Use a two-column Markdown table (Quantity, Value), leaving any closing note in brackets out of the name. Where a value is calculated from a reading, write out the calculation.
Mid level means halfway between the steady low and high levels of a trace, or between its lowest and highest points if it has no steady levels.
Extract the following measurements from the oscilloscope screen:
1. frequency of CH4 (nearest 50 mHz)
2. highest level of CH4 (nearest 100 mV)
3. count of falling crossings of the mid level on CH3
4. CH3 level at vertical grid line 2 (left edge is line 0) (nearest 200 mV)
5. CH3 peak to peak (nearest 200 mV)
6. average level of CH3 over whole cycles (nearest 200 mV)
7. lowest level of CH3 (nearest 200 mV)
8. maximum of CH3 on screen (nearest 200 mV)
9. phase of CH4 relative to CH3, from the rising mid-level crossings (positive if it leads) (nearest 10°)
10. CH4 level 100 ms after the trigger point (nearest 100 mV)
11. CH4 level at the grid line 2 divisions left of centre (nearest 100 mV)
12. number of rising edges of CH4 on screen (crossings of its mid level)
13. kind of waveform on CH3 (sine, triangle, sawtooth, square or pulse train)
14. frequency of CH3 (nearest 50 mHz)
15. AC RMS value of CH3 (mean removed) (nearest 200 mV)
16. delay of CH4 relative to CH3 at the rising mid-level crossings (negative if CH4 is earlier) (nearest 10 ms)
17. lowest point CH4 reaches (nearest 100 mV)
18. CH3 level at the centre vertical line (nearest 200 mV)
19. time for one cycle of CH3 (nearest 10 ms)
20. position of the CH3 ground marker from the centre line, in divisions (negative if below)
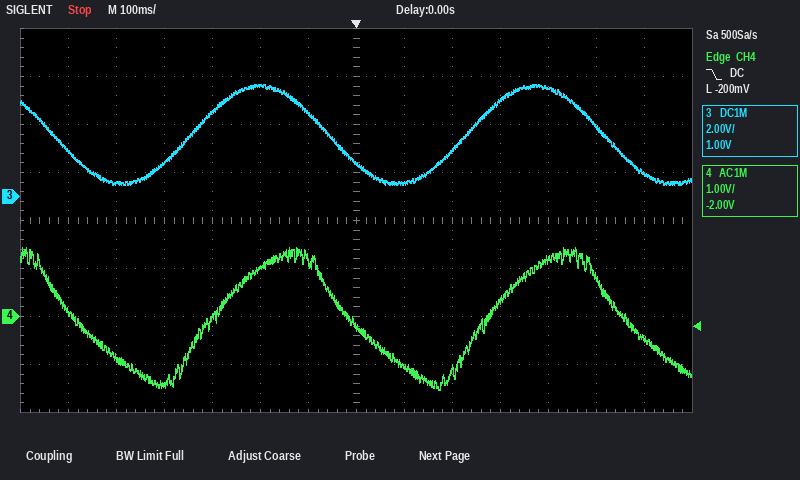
| Quantity | Value |
|---|---|
| frequency of CH4 | 1.75 Hz |
| highest level of CH4 | 1.4 V |
| count of falling crossings of the mid level on CH3 | 3 |
| CH3 level at vertical grid line 2 (left edge is line 0) | 600 mV |
| CH3 peak to peak | 4.6 V − (400 mV) = 4.2 V |
| average level of CH3 over whole cycles | (4.6 V + (400 mV)) / 2 ≈ 2.50 V, so 2.6 V to the nearest 200 mV |
| lowest level of CH3 | 400 mV |
| maximum of CH3 on screen | 4.6 V |
| phase of CH4 relative to CH3, from the rising mid-level crossings (positive if it leads) | −360° × (+40 ms) / 570 ms ≈ -25.3°, so -30° to the nearest 10° |
| CH4 level 100 ms after the trigger point | -1.0 V |
| CH4 level at the grid line 2 divisions left of centre | 1.0 V |
| number of rising edges of CH4 on screen | 2 |
| kind of waveform on CH3 | sine |
| frequency of CH3 | 1 / 570 ms ≈ 1.75 Hz |
| AC RMS value of CH3 (mean removed) | 4.2 V / (2√2) ≈ 1.48 V, so 1.4 V to the nearest 200 mV |
| delay of CH4 relative to CH3 at the rising mid-level crossings (negative if CH4 is earlier) | +40 ms |
| lowest point CH4 reaches | -1.5 V |
| CH3 level at the centre vertical line | 1.4 V |
| time for one cycle of CH3 | 570 ms |
| position of the CH3 ground marker from the centre line, in divisions | +0.5 div |
